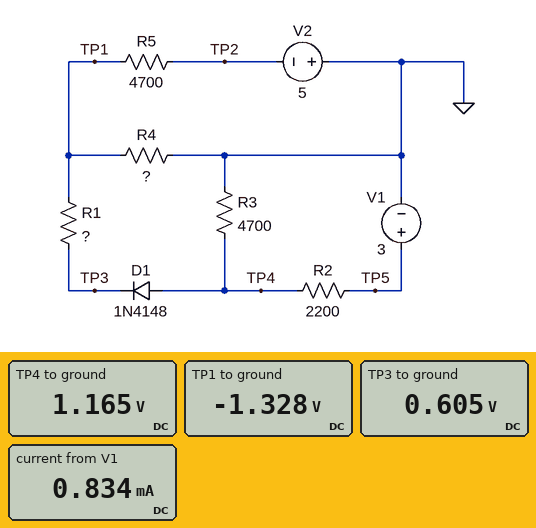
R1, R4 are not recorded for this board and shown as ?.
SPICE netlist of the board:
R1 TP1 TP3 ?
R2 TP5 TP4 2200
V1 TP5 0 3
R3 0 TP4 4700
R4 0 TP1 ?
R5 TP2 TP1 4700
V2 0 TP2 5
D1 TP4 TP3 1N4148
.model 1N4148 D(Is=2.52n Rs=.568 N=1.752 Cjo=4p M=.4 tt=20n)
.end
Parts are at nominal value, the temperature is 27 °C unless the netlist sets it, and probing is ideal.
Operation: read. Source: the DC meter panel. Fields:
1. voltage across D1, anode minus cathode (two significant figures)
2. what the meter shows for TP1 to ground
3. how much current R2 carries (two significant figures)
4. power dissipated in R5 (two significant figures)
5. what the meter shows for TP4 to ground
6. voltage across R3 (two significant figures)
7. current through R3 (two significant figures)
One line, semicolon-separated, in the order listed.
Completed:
560 mV; -1.328 V; 830 µA; 2.9 mW; 1.165 V; 1.2 V; 250 µA
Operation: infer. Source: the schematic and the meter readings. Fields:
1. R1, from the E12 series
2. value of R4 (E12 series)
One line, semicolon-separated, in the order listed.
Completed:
3.3 kΩ; 6.8 kΩ
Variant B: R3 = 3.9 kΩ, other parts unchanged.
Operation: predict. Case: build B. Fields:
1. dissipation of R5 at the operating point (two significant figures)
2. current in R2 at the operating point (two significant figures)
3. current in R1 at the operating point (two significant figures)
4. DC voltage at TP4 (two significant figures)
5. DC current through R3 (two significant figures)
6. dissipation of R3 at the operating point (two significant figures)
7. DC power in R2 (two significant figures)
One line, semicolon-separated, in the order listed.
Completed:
2.8 mW; 860 µA; 580 µA; 1.1 V; 280 µA; 310 µW; 1.6 mW
